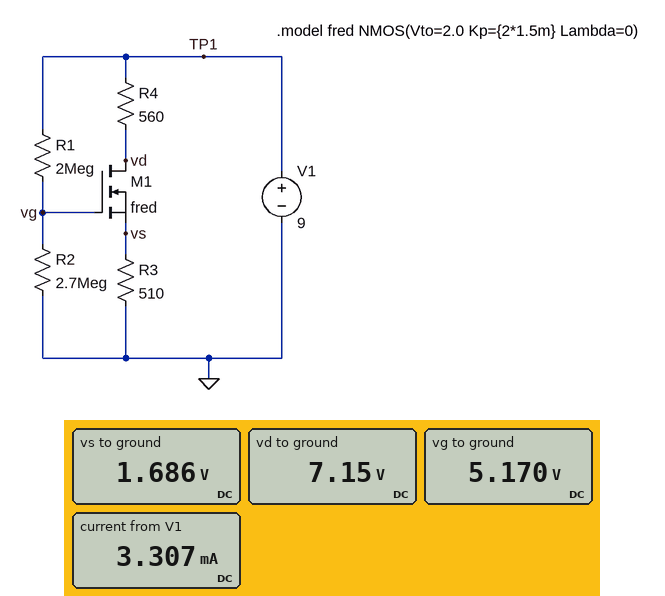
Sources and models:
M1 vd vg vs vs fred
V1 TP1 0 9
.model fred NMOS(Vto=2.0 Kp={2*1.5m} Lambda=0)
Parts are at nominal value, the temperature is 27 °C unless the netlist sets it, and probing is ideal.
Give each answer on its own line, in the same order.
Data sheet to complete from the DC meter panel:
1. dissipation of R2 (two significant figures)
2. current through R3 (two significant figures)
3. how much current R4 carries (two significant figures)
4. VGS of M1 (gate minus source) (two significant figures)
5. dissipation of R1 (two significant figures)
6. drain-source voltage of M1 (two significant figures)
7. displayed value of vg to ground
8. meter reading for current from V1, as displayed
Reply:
9.9 µW
3.3 mA
3.3 mA
3.5 V
7.3 µW
5.5 V
5.170 V
3.307 mA
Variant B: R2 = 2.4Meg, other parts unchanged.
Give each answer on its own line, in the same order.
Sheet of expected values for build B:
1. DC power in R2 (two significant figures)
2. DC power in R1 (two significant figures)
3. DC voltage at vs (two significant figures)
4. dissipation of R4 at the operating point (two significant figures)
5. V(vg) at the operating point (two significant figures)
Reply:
10 µW
8.4 µW
1.5 V
4.9 mW
4.9 V
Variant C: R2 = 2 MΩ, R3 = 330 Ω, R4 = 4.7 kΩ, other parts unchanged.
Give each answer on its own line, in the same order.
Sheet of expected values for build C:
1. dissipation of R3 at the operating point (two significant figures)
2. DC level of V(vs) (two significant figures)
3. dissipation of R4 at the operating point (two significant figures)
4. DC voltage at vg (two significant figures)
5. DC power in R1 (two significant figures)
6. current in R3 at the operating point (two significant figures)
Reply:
980 µW
570 mV
14 mW
4.5 V
10 µW
1.7 mA
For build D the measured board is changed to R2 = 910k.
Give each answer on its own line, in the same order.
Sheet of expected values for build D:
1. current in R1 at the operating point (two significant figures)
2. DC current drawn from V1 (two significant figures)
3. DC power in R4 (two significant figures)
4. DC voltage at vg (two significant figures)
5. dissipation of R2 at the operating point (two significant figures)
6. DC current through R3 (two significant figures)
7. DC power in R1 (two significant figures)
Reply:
3.1 µA
490 µA
130 µW
2.8 V
8.7 µW
480 µA
19 µW
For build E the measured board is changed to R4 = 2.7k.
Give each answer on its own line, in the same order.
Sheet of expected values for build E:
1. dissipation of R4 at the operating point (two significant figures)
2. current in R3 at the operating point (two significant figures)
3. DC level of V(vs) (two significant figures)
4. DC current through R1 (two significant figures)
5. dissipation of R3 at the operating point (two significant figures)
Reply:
19 mW
2.6 mA
1.3 V
1.9 µA
3.5 mW
